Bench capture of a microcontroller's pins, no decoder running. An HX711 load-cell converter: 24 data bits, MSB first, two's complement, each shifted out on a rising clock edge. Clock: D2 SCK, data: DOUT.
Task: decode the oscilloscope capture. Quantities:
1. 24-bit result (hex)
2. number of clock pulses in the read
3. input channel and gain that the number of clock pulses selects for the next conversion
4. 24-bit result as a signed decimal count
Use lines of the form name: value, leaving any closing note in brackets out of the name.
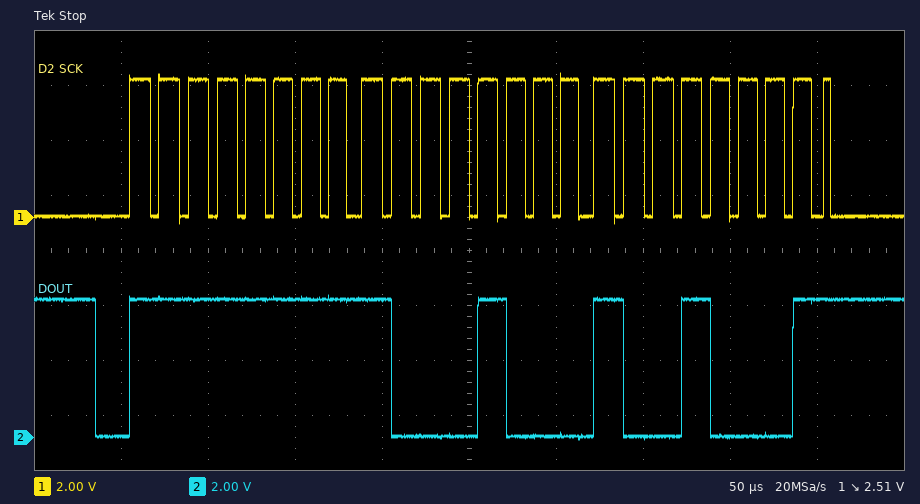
24-bit result: 0xFF8891
number of clock pulses in the read: 25
input channel and gain that the number of clock pulses selects for the next conversion: channel A, gain 128
24-bit result as a signed decimal count: -30575
